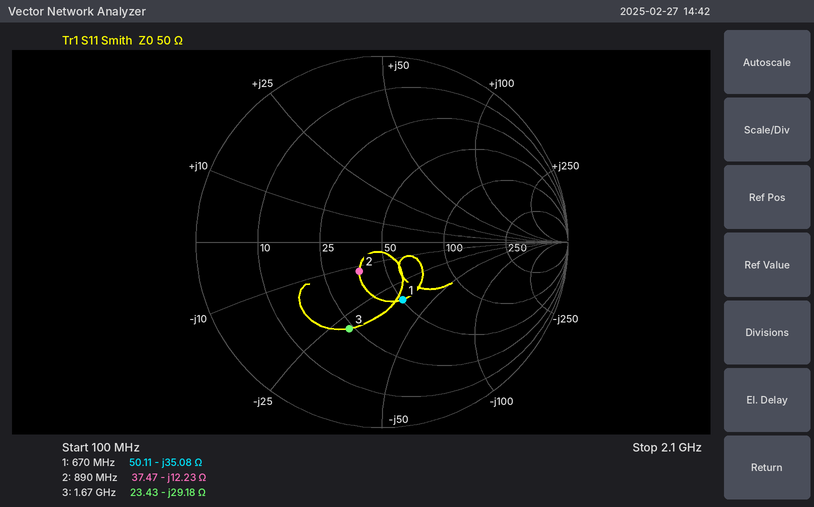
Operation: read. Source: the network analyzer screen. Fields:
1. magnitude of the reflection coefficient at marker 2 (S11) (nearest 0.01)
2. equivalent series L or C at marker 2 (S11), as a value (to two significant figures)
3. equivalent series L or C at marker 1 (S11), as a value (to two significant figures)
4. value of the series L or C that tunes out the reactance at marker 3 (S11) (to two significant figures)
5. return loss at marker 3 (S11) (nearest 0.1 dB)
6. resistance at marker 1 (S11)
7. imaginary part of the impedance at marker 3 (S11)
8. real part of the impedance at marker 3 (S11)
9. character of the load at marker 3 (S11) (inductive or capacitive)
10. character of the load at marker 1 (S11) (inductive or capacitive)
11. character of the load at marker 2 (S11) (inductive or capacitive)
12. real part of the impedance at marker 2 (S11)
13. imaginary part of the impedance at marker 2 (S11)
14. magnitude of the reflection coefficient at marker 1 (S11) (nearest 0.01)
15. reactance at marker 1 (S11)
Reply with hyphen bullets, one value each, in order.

- 0.20
- 15 pF
- 6.8 pF
- 2.8 nH
- 6.0 dB
- 50.11 Ω
- -29.18 Ω
- 23.43 Ω
- capacitive
- capacitive
- capacitive
- 37.47 Ω
- -12.23 Ω
- 0.33
- -35.08 Ω
